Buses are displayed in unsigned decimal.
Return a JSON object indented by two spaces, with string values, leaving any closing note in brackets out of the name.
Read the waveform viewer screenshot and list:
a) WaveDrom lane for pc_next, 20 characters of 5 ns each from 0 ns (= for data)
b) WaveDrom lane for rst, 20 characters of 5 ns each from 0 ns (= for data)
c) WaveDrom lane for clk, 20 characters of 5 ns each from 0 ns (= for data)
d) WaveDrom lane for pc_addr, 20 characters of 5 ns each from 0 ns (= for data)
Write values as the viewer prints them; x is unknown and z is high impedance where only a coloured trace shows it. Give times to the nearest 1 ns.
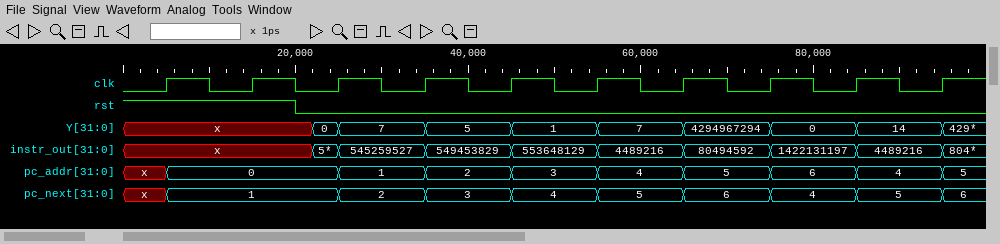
{
  "WaveDrom lane for pc_next, 20 characters of 5 ns each from 0 ns": "{name: 'pc_next', wave: 'x=...=.=.=.=.=.=.=.=', data: '1 2 3 4 5 6 4 5 6'}",
  "WaveDrom lane for rst, 20 characters of 5 ns each from 0 ns": "{name: 'rst', wave: '1...0...............'}",
  "WaveDrom lane for clk, 20 characters of 5 ns each from 0 ns": "{name: 'clk', wave: '01010101010101010101'}",
  "WaveDrom lane for pc_addr, 20 characters of 5 ns each from 0 ns": "{name: 'pc_addr', wave: 'x=...=.=.=.=.=.=.=.=', data: '0 1 2 3 4 5 6 4 5'}"
}
